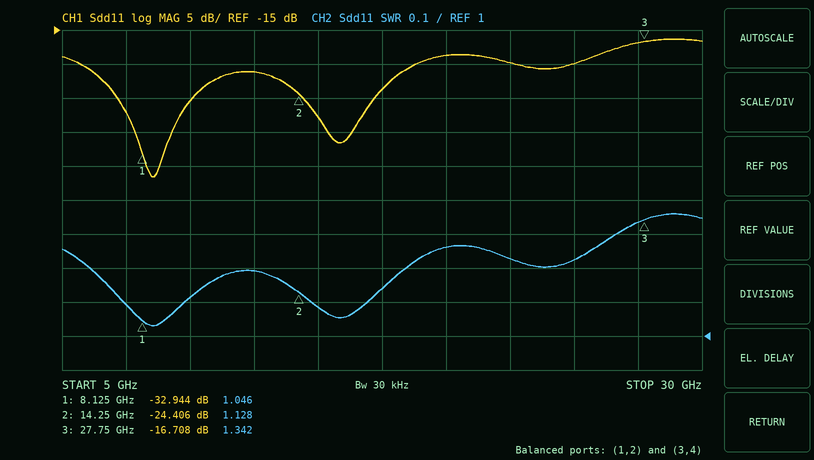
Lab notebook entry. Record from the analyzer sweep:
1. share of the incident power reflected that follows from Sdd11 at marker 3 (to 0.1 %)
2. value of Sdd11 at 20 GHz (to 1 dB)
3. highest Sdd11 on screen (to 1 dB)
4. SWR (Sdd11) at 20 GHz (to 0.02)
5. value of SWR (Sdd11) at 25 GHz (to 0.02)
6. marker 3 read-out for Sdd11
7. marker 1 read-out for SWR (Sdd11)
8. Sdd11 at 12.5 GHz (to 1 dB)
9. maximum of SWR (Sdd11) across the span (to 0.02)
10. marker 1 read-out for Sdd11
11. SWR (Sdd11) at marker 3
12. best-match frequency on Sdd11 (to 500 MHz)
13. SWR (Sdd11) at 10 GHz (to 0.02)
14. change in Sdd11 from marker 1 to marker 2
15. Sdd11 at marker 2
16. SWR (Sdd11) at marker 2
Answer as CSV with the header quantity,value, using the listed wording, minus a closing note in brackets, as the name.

quantity,value
share of the incident power reflected that follows from Sdd11 at marker 3,2.1 %
value of Sdd11 at 20 GHz,-19 dB
highest Sdd11 on screen,-16 dB
SWR (Sdd11) at 20 GHz,1.26
value of SWR (Sdd11) at 25 GHz,1.22
marker 3 read-out for Sdd11,-16.708 dB
marker 1 read-out for SWR,1.046
Sdd11 at 12.5 GHz,-21 dB
maximum of SWR (Sdd11) across the span,1.36
marker 1 read-out for Sdd11,-32.944 dB
SWR (Sdd11) at marker 3,1.342
best-match frequency on Sdd11,8.5 GHz
SWR (Sdd11) at 10 GHz,1.12
change in Sdd11 from marker 1 to marker 2,8.538 dB
Sdd11 at marker 2,-24.406 dB
SWR (Sdd11) at marker 2,1.128
